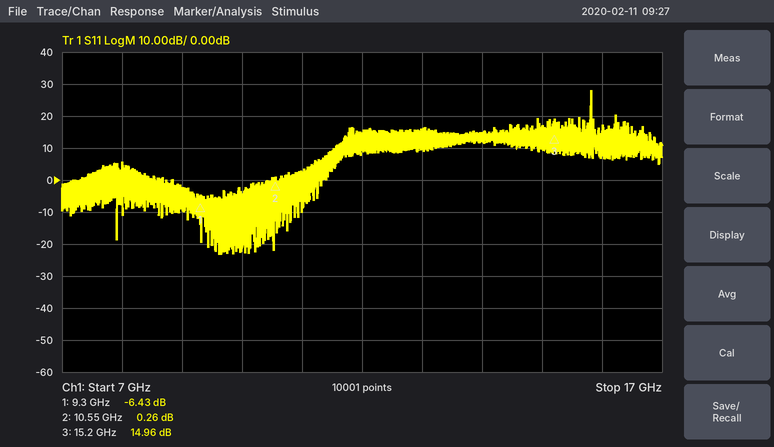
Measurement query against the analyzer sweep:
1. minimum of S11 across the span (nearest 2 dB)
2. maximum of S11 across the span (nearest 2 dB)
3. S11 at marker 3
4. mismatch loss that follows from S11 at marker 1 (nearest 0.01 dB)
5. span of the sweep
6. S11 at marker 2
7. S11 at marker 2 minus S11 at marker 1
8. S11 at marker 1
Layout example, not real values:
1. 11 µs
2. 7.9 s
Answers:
1. -24 dB
2. 28 dB
3. 14.96 dB
4. 1.12 dB
5. 10 GHz
6. 0.26 dB
7. 6.69 dB
8. -6.43 dB
